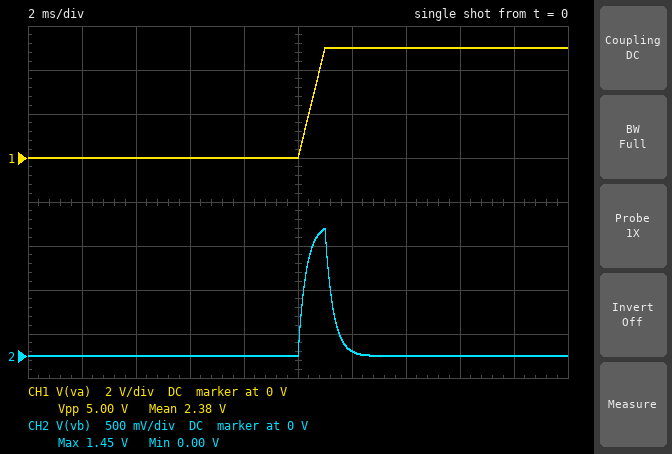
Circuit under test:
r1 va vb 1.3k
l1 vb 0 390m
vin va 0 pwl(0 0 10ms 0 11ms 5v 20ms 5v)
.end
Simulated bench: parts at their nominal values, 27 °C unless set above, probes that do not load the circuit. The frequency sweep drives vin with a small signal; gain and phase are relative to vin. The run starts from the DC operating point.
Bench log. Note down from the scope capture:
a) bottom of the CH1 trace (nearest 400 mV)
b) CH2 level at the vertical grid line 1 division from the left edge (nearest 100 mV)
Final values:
0 V
0 V
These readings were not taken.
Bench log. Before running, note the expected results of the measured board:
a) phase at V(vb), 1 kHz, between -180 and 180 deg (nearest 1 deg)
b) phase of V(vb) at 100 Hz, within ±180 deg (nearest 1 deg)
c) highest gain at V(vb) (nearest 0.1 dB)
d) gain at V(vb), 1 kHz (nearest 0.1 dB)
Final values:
28 deg
79 deg
0 dB
-1.1 dB
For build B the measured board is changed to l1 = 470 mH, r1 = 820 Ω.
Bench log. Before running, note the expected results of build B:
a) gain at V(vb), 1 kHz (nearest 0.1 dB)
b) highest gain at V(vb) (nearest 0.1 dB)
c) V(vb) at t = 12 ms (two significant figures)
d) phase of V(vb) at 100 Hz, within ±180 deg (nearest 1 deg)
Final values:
-0.3 dB
0 dB
410 mV
70 deg
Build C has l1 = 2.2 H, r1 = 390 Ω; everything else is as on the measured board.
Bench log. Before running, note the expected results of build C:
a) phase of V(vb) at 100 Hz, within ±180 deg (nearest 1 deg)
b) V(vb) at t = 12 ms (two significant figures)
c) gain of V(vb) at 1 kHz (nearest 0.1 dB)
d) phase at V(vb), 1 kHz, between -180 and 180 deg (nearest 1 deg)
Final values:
16 deg
3.8 V
0 dB
2 deg
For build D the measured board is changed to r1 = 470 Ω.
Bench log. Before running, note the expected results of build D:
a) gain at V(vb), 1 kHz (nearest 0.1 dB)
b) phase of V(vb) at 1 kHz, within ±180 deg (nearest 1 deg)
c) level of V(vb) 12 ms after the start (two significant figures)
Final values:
-0.2 dB
11 deg
870 mV
